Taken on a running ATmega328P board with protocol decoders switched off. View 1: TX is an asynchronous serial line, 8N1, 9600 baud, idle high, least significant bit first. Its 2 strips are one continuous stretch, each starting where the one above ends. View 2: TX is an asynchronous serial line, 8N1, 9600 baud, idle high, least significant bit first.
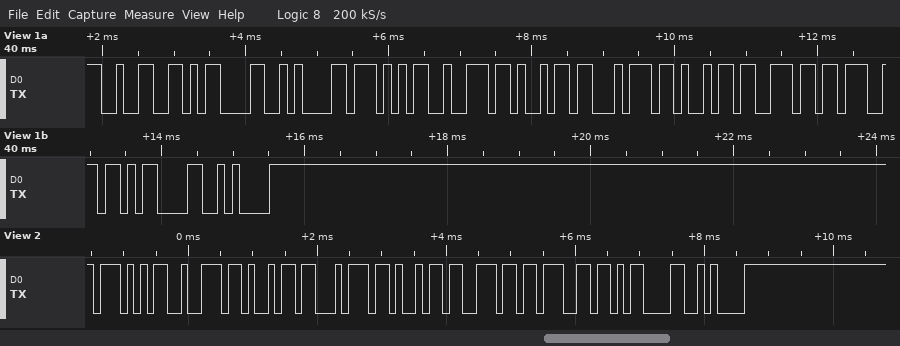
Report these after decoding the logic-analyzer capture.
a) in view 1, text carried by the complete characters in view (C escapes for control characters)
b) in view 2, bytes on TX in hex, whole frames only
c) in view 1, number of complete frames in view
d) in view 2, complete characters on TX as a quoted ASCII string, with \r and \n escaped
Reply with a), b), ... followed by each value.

a) "2\r\nWriting\r\n"
b) 57 72 69 74 69 6E 67 0D 0A
c) 12
d) "Writing\r\n"
